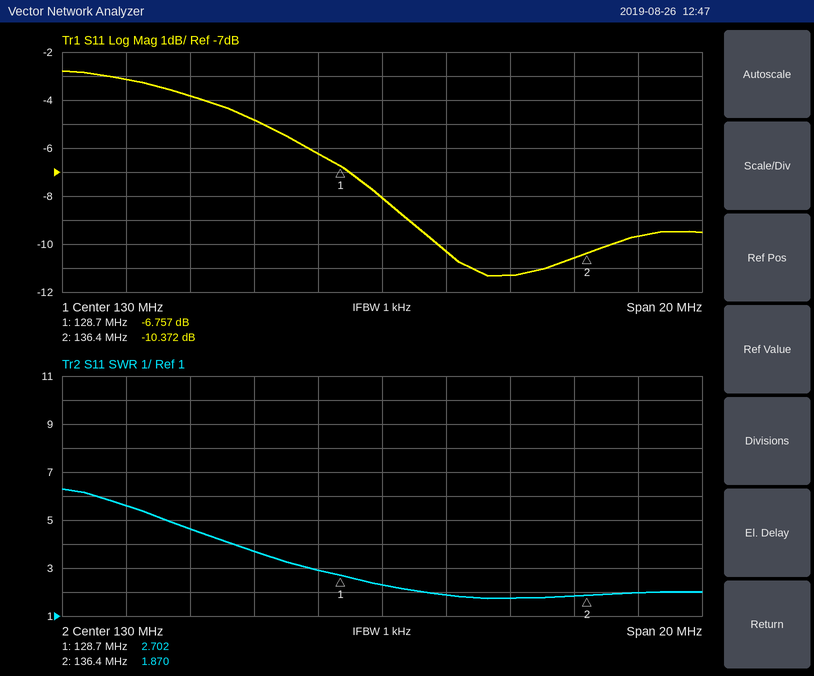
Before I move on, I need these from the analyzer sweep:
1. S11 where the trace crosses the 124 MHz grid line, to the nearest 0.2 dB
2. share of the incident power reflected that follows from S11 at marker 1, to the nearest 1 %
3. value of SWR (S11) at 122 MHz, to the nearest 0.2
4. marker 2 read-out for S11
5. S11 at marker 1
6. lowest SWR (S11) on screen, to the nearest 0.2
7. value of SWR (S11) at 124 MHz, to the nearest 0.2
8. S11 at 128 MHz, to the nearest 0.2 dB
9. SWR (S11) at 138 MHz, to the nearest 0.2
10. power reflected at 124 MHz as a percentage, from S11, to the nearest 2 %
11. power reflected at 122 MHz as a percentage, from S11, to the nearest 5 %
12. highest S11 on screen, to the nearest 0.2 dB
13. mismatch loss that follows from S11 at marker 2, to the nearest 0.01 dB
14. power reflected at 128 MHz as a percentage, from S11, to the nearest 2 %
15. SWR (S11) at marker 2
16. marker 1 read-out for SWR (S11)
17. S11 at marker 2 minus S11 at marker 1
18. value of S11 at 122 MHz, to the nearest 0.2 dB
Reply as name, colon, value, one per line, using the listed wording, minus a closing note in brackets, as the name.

S11 where the trace crosses the 124 MHz grid line, to the nearest 0.2 dB: -3.8 dB
share of the incident power reflected that follows from S11 at marker 1, to the nearest 1 %: 21 %
value of SWR (S11) at 122 MHz, to the nearest 0.2: 5.6
marker 2 read-out for S11: -10.372 dB
S11 at marker 1: -6.757 dB
lowest SWR (S11) on screen, to the nearest 0.2: 1.8
value of SWR (S11) at 124 MHz, to the nearest 0.2: 4.6
S11 at 128 MHz, to the nearest 0.2 dB: -6.2 dB
SWR (S11) at 138 MHz, to the nearest 0.2: 2.0
power reflected at 124 MHz as a percentage, from S11, to the nearest 2 %: 42 %
power reflected at 122 MHz as a percentage, from S11, to the nearest 5 %: 50 %
highest S11 on screen, to the nearest 0.2 dB: -2.8 dB
mismatch loss that follows from S11 at marker 2, to the nearest 0.01 dB: 0.42 dB
power reflected at 128 MHz as a percentage, from S11, to the nearest 2 %: 24 %
SWR (S11) at marker 2: 1.870
marker 1 read-out for SWR: 2.702
S11 at marker 2 minus S11 at marker 1: -3.615 dB
value of S11 at 122 MHz, to the nearest 0.2 dB: -3.2 dB
